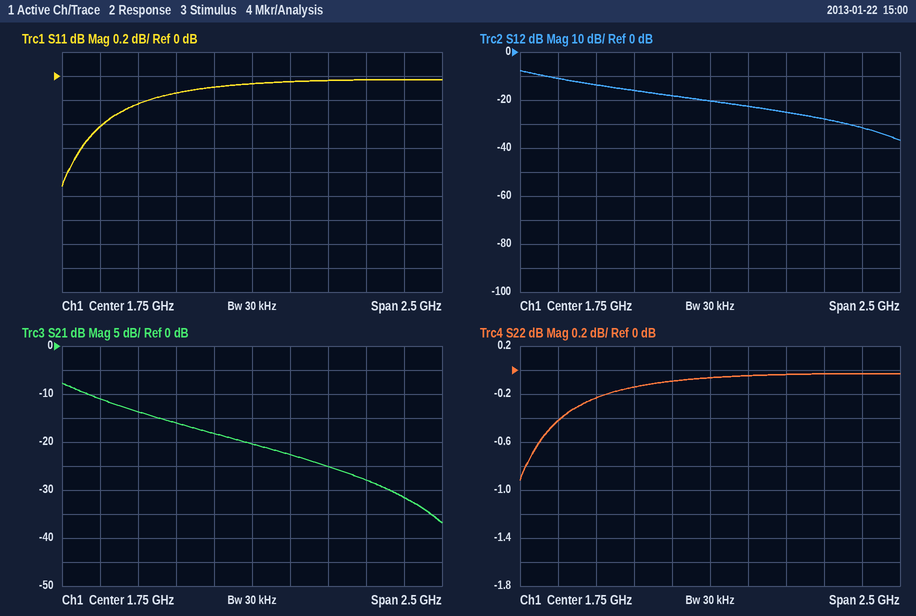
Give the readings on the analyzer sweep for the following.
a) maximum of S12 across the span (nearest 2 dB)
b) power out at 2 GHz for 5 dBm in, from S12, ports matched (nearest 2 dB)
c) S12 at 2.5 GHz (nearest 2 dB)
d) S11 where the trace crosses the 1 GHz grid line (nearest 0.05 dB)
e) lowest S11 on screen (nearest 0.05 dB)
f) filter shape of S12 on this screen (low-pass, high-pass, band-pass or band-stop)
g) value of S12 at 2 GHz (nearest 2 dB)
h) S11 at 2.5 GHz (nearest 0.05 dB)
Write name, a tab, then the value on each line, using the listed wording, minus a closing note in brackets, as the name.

maximum of S12 across the span	-8 dB
power out at 2 GHz for 5 dBm in, from S12, ports matched	-18 dBm
S12 at 2.5 GHz	-28 dB
S11 where the trace crosses the 1 GHz grid line	-0.25 dB
lowest S11 on screen	-0.90 dB
filter shape of S12 on this screen	low-pass
value of S12 at 2 GHz	-22 dB
S11 at 2.5 GHz	-0.05 dB
